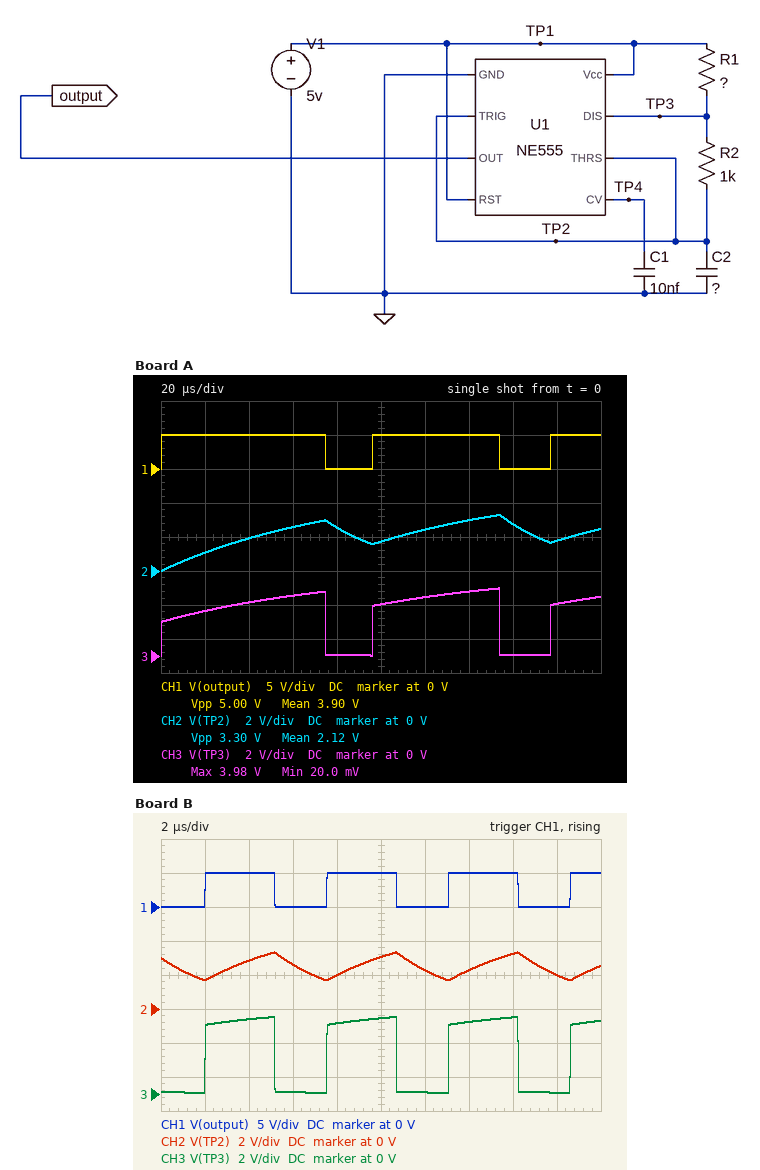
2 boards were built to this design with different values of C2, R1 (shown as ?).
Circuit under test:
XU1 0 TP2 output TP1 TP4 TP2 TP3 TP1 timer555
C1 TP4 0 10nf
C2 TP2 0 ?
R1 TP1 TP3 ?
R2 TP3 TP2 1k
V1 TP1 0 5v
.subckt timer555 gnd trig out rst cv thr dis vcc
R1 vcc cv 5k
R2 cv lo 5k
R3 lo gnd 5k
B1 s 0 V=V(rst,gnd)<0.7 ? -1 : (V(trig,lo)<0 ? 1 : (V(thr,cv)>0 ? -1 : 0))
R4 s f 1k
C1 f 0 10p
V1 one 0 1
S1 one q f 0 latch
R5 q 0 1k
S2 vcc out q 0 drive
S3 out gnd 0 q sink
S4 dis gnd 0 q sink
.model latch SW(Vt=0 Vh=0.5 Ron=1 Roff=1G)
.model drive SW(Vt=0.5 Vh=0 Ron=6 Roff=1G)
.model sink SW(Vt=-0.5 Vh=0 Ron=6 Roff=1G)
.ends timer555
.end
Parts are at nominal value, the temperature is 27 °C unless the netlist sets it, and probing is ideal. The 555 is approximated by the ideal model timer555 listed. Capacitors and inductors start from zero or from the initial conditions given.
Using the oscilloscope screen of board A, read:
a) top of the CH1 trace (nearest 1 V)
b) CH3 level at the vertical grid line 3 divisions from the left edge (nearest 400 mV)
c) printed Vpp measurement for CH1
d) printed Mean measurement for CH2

5 V
3.6 V
5.00 V
2.12 V
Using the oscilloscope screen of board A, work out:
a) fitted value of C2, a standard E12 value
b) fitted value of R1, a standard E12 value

33 nF
1.5 kΩ
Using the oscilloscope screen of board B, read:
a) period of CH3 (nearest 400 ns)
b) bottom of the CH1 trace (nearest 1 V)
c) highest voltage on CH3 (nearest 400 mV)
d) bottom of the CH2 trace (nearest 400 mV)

5.6 µs
0 V
4.4 V
1.6 V
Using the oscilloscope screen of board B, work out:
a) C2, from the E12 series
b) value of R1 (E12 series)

3.3 nF
390 Ω
